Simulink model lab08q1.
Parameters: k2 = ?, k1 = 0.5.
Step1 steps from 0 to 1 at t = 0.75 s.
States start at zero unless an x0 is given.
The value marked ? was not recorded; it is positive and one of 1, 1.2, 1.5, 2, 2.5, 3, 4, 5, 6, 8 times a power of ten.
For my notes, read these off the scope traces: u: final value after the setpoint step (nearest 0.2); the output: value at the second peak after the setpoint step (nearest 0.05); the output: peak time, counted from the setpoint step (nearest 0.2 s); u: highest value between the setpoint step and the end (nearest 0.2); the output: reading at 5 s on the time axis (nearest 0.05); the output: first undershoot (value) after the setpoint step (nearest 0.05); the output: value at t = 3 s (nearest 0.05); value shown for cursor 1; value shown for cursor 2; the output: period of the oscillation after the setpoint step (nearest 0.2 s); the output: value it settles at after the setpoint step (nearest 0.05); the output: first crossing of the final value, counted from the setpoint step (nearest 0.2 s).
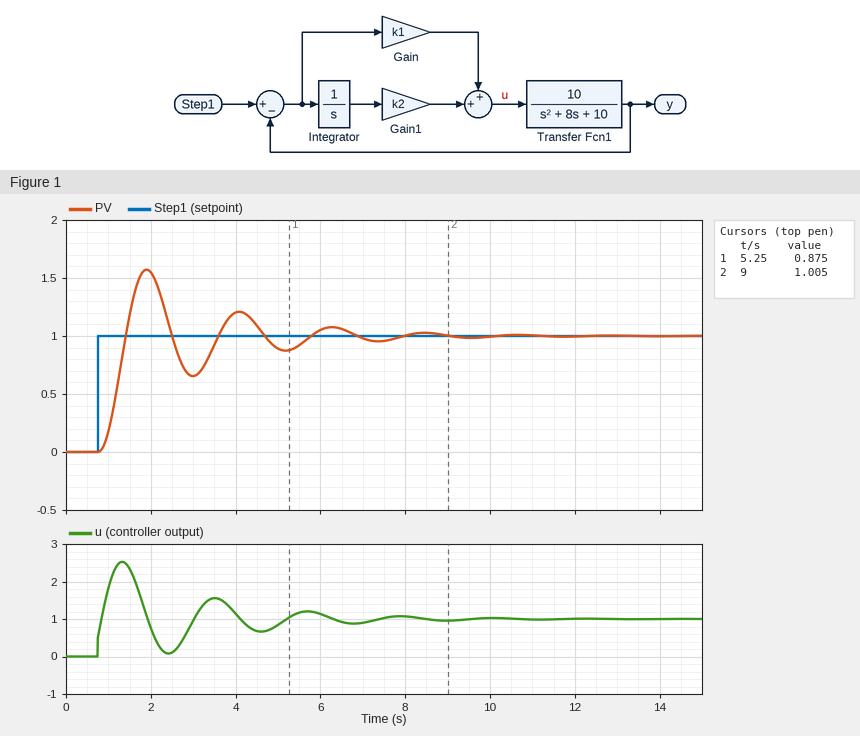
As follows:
1.0
1.20
1.2 s
2.6
0.90
0.65
0.65
0.875
1.005
2.2 s
1.00
0.6 s
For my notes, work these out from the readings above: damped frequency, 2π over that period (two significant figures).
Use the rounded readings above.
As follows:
2.9 rad/s
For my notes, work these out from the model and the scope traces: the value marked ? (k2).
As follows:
6
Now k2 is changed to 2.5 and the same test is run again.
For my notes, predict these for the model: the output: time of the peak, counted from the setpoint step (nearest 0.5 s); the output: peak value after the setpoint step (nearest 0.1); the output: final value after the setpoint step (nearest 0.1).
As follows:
1.5 s
1.2
1.0
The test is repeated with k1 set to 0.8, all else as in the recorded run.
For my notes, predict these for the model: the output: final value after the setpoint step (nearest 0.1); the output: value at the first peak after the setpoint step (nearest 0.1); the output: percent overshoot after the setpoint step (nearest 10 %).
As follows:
1.0
1.5
50 %
